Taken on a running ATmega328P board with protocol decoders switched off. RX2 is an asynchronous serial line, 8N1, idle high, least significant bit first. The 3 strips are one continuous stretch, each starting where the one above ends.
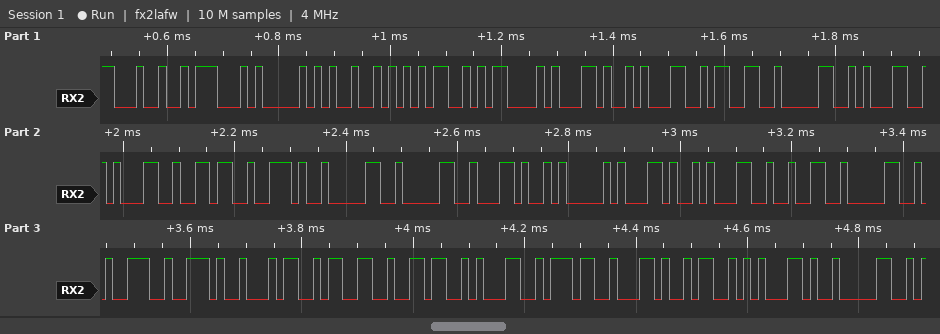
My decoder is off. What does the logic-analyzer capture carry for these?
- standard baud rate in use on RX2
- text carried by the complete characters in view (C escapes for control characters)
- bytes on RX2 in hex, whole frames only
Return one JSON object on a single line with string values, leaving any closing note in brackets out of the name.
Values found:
{"standard baud rate in use on RX2": "74880 baud", "text carried by the complete characters in view": "\"$GPRMC,130116.00,A,1209.43617,S,0\"", "bytes on RX2 in hex, whole frames only": "0x24 0x47 0x50 0x52 0x4D 0x43 0x2C 0x31 0x33 0x30 0x31 0x31 0x36 0x2E 0x30 0x30 0x2C 0x41 0x2C 0x31 0x32 0x30 0x39 0x2E 0x34 0x33 0x36 0x31 0x37 0x2C 0x53 0x2C 0x30"}
